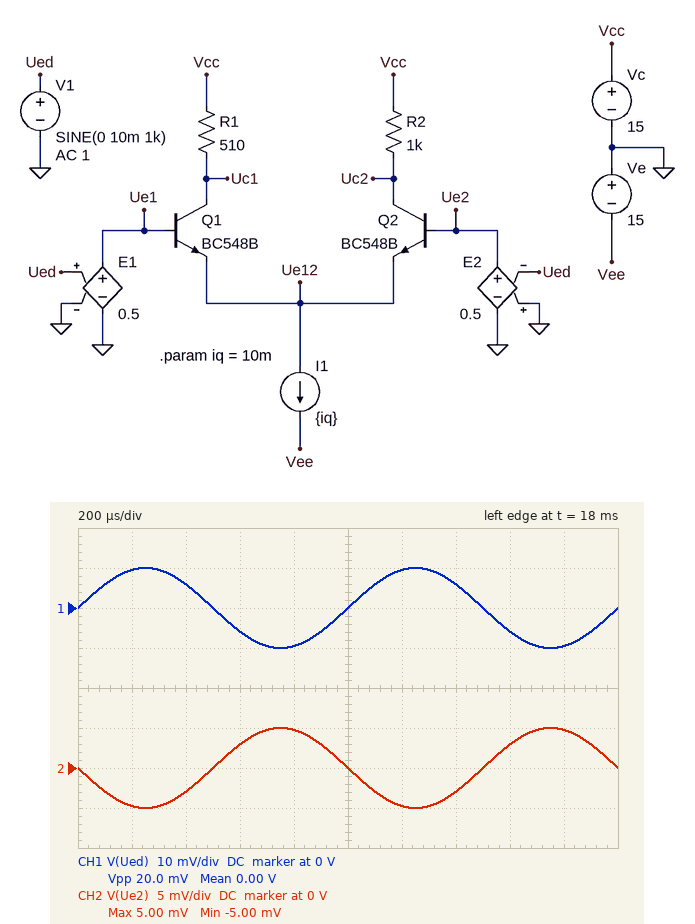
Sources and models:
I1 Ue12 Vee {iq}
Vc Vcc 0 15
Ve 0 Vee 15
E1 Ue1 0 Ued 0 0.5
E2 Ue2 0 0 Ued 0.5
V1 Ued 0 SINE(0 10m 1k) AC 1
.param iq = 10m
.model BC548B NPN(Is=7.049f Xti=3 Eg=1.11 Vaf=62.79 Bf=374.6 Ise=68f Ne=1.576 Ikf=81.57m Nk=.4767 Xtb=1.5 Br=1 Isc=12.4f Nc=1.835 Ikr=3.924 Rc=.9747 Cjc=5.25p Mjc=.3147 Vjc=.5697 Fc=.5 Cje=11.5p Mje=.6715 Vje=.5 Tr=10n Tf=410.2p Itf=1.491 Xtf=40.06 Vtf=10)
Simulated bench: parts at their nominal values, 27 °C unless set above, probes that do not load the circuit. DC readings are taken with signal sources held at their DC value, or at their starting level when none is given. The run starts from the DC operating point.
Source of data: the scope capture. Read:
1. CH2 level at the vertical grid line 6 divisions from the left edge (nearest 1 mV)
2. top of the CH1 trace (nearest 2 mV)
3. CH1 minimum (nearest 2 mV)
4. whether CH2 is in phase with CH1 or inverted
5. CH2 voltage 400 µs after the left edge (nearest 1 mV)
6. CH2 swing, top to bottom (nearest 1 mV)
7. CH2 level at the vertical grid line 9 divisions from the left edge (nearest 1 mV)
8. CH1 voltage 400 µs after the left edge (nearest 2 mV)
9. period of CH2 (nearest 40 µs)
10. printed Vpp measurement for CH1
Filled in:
-5 mV
10 mV
-10 mV
inverted
-3 mV
10 mV
5 mV
6 mV
1.00 ms
20.0 mV
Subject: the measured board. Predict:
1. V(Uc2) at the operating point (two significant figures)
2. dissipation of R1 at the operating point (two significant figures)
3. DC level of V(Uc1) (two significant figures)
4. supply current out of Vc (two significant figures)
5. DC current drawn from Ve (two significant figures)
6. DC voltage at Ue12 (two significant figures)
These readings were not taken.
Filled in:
10 V
13 mW
12 V
10 mA
10 mA
-700 mV
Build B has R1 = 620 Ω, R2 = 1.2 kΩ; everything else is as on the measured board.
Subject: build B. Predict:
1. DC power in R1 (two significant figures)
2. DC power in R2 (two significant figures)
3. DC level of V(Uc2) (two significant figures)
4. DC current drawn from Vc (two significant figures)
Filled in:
16 mW
29 mW
9.1 V
10 mA
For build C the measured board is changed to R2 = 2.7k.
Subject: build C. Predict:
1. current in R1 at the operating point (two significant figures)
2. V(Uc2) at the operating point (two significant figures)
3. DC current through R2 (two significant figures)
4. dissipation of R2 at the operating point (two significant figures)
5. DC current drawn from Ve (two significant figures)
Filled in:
5.3 mA
2.5 V
4.6 mA
58 mW
10 mA
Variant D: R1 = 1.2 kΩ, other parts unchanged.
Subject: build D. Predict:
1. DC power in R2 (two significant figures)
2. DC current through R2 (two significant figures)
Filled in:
25 mW
5.0 mA
